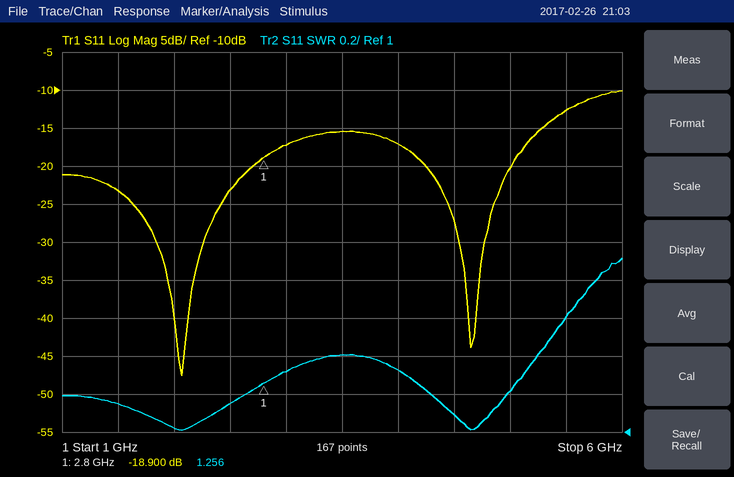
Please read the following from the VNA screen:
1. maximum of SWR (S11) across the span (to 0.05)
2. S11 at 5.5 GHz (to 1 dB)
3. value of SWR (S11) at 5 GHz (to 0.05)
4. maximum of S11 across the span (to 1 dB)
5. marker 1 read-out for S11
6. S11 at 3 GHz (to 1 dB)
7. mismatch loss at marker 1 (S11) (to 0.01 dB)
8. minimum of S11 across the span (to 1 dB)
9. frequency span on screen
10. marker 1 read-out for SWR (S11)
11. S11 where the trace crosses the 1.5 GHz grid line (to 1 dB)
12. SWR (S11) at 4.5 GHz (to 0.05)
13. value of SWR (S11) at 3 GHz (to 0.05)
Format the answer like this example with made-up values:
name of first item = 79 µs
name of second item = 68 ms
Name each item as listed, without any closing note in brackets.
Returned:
maximum of SWR (S11) across the span = 1.90
S11 at 5.5 GHz = -13 dB
value of SWR (S11) at 5 GHz = 1.20
maximum of S11 across the span = -10 dB
marker 1 read-out for S11 = -18.900 dB
S11 at 3 GHz = -17 dB
mismatch loss at marker 1 (S11) = 0.06 dB
minimum of S11 across the span = -48 dB
frequency span on screen = 5 GHz
marker 1 read-out for SWR = 1.256
S11 where the trace crosses the 1.5 GHz grid line = -23 dB
SWR (S11) at 4.5 GHz = 1.10
value of SWR (S11) at 3 GHz = 1.30
